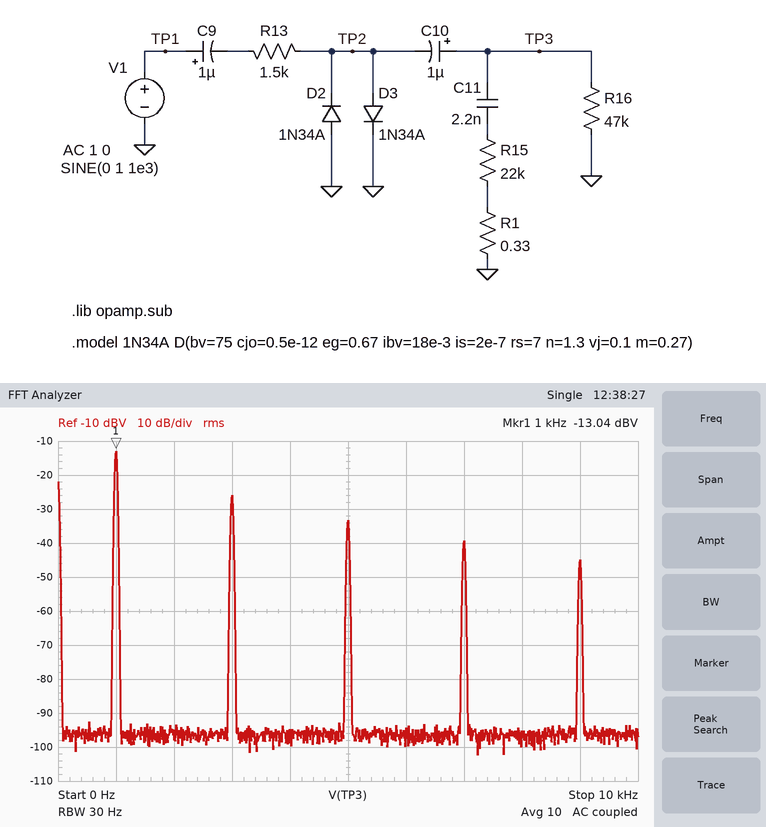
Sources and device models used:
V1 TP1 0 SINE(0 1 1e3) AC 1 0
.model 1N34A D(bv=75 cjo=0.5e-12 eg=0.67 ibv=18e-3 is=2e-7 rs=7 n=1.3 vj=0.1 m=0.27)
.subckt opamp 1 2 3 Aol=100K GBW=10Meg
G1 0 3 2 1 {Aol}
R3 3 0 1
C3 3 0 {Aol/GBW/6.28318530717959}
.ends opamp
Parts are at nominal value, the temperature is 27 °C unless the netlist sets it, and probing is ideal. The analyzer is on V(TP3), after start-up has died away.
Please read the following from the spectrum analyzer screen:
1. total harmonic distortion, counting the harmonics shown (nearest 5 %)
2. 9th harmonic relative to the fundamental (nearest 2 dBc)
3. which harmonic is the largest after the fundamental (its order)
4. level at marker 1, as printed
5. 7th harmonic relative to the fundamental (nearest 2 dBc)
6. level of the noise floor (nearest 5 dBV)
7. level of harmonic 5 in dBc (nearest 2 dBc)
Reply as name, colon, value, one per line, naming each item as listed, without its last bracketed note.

total harmonic distortion, counting the harmonics shown: 25 %
9th harmonic relative to the fundamental: -32 dBc
which harmonic is the largest after the fundamental: 3
level at marker 1, as printed: -13.04 dBV
7th harmonic relative to the fundamental: -26 dBc
level of the noise floor: -95 dBV
level of harmonic 5 in dBc: -20 dBc
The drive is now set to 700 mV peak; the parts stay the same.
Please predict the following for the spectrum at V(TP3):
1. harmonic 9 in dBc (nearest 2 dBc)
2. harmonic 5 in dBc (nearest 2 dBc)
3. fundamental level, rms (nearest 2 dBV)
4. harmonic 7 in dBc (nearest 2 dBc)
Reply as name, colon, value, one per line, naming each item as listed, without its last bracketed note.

harmonic 9 in dBc: -40 dBc
harmonic 5 in dBc: -22 dBc
fundamental level, rms: -14 dBV
harmonic 7 in dBc: -30 dBc
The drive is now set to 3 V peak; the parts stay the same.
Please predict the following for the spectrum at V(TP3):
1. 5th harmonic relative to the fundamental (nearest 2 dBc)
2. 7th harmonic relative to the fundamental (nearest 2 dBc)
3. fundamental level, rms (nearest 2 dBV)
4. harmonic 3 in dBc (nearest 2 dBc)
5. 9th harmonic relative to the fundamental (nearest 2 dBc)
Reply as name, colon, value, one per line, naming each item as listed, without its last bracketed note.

5th harmonic relative to the fundamental: -18 dBc
7th harmonic relative to the fundamental: -22 dBc
fundamental level, rms: -12 dBV
harmonic 3 in dBc: -12 dBc
9th harmonic relative to the fundamental: -24 dBc
